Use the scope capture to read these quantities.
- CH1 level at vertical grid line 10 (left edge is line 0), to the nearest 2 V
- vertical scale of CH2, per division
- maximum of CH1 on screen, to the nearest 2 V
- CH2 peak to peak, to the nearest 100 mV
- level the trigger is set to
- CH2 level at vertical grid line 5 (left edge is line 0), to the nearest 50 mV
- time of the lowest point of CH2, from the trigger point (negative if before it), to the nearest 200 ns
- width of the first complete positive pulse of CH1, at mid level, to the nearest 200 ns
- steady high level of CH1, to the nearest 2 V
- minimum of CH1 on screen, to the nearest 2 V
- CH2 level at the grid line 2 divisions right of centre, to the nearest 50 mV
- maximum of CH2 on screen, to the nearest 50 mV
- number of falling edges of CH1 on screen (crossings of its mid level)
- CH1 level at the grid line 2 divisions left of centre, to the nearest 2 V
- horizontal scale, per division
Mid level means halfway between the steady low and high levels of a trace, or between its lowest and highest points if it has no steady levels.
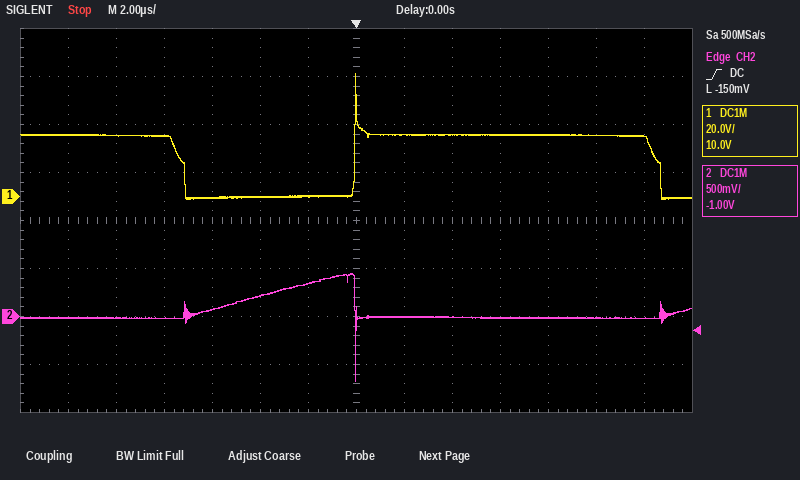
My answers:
26 V
500 mV
52 V
1.10 V
-150 mV
200 mV
0.0 µs
12.8 µs
26 V
-2 V
0 mV
450 mV
2
0 V
2 µs
